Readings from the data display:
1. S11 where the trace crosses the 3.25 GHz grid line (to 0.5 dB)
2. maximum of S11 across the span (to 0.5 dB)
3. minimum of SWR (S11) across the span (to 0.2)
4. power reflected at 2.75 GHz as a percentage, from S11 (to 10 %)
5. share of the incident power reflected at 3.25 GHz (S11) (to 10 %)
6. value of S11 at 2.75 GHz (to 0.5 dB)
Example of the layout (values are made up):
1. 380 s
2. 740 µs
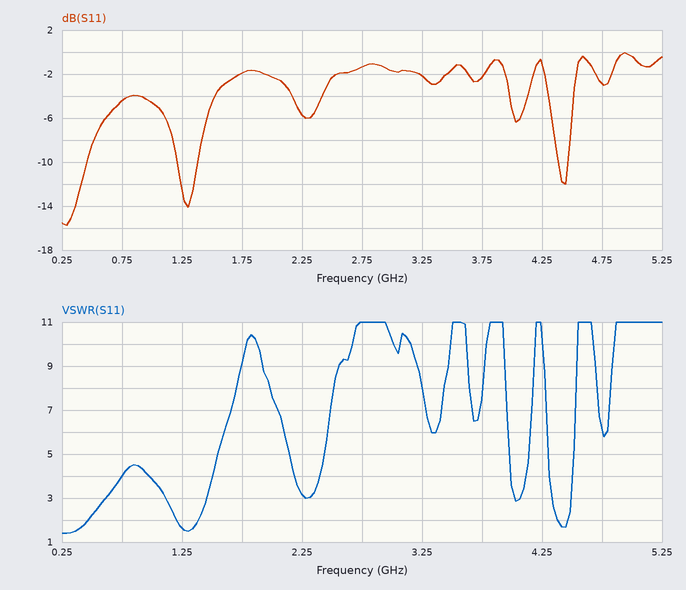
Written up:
1. -2.0 dB
2. 0.0 dB
3. 1.4
4. 70 %
5. 60 %
6. -1.5 dB
